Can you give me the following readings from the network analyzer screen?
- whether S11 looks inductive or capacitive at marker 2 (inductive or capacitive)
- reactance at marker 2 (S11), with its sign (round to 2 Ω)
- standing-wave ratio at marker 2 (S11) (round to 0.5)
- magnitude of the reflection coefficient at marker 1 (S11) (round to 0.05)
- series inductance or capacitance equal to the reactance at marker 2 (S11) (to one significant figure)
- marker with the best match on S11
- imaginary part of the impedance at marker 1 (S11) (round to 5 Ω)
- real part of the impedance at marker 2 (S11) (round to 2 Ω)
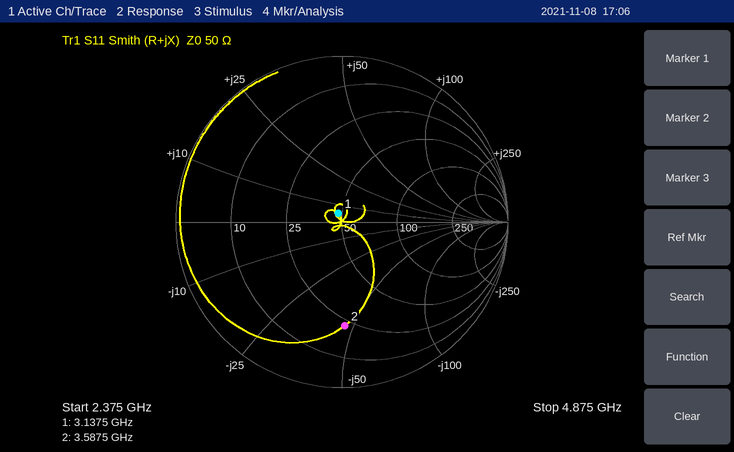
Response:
capacitive
-46 Ω
4.5
0.05
1.0 pF
marker 1
+5 Ω
22 Ω
